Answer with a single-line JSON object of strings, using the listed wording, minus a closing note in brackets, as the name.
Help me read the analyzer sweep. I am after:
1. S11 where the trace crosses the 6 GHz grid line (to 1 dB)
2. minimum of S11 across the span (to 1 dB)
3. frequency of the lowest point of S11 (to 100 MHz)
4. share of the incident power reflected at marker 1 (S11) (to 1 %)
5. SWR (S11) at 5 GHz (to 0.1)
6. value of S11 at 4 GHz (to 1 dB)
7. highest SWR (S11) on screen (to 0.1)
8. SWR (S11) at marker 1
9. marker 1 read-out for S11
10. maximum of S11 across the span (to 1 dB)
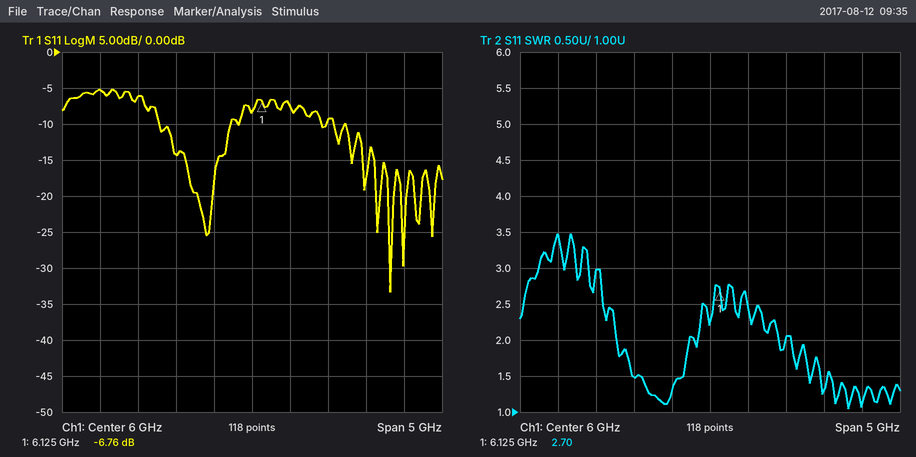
{"S11 where the trace crosses the 6 GHz grid line": "-8 dB", "minimum of S11 across the span": "-33 dB", "frequency of the lowest point of S11": "7.8 GHz", "share of the incident power reflected at marker 1 (S11)": "21 %", "SWR (S11) at 5 GHz": "1.5", "value of S11 at 4 GHz": "-5 dB", "highest SWR (S11) on screen": "3.5", "SWR (S11) at marker 1": "2.70", "marker 1 read-out for S11": "-6.76 dB", "maximum of S11 across the span": "-5 dB"}
